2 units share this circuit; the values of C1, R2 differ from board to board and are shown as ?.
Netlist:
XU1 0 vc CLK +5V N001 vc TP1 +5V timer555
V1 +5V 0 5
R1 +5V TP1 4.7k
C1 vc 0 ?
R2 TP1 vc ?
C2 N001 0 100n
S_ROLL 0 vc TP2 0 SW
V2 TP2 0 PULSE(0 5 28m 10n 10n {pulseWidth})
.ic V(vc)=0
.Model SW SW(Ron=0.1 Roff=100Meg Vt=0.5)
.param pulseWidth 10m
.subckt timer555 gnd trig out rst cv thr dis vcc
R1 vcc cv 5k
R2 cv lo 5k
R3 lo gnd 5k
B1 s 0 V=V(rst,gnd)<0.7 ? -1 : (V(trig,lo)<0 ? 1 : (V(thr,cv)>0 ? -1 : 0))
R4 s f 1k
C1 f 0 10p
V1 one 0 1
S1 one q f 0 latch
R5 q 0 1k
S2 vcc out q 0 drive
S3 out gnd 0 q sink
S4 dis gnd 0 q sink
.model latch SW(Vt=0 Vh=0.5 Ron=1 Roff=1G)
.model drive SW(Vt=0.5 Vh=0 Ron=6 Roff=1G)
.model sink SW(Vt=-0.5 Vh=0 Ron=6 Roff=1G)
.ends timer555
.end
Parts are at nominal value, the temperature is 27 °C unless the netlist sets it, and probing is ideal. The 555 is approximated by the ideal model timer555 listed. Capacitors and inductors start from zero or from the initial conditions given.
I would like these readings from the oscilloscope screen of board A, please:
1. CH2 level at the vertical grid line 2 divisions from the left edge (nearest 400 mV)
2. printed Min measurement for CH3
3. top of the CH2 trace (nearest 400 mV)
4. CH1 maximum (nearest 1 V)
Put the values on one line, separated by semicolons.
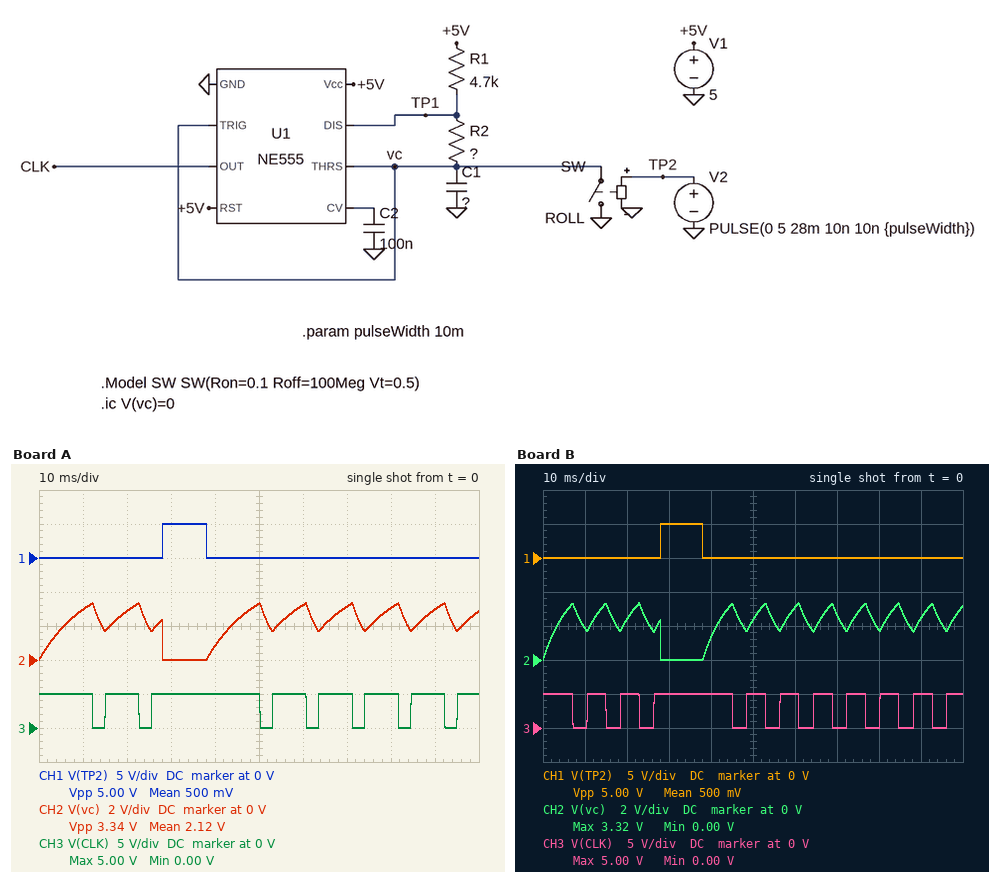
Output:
2.8 V; 0.00 V; 3.2 V; 5 V
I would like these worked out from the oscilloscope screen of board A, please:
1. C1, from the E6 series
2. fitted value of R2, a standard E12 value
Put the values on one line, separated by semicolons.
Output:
1.5 µF; 2.7 kΩ
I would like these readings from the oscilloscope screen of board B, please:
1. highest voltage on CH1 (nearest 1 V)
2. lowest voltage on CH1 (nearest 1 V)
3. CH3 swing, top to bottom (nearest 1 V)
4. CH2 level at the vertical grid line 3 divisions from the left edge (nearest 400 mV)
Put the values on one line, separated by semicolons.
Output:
5 V; 0 V; 5 V; 0 V
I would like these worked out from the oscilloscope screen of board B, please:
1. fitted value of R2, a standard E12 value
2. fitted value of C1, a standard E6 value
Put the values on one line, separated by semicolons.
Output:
15 kΩ; 330 nF
